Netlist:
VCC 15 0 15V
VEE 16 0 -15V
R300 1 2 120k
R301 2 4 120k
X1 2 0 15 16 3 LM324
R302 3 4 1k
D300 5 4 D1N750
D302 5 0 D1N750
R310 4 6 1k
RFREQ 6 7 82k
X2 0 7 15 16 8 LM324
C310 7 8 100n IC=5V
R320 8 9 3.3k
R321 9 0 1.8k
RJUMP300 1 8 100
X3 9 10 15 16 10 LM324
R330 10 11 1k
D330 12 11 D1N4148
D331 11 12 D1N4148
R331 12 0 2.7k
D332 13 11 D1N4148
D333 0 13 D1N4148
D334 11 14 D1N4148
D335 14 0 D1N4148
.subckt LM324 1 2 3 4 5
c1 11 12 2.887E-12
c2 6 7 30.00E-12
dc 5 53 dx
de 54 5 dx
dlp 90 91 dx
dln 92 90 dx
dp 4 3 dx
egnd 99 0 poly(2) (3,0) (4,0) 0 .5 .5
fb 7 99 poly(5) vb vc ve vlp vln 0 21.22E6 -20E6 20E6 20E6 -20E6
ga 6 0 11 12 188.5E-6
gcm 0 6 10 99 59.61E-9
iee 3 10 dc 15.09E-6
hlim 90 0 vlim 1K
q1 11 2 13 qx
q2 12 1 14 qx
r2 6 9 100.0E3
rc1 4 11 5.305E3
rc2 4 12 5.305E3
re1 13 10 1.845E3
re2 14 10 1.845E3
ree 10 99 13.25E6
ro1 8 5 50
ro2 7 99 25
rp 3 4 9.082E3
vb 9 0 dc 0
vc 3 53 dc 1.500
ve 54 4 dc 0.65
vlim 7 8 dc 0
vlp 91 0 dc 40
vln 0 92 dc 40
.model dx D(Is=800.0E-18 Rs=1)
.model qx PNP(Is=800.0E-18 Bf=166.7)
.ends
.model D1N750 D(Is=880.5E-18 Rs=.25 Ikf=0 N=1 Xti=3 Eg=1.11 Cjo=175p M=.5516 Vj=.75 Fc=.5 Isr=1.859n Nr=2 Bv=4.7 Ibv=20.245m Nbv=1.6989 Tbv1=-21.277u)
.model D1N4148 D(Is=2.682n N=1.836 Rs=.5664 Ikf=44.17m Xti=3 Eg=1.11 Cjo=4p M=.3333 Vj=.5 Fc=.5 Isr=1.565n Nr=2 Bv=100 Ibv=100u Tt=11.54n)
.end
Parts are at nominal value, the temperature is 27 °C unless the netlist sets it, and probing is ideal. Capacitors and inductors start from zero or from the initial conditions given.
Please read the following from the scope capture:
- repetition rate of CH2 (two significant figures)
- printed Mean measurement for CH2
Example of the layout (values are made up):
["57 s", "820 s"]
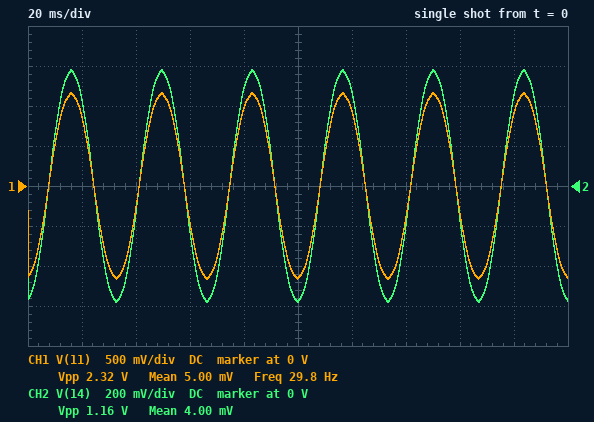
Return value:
["30 Hz", "4.00 mV"]
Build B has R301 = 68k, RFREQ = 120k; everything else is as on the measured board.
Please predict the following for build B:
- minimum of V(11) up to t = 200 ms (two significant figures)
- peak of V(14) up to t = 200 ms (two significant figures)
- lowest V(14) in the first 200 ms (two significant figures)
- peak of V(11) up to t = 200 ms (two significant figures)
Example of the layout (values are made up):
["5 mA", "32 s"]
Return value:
["-1.3 V", "640 mV", "-640 mV", "1.3 V"]
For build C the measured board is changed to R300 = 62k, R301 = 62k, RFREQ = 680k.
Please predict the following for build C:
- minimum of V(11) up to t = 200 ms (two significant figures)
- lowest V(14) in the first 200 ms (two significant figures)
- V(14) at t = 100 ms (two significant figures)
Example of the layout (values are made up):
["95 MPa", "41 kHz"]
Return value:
["-1.1 V", "-570 mV", "440 mV"]
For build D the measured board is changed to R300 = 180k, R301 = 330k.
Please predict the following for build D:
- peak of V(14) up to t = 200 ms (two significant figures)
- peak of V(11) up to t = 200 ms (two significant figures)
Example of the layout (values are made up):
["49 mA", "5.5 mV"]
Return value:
["440 mV", "890 mV"]
